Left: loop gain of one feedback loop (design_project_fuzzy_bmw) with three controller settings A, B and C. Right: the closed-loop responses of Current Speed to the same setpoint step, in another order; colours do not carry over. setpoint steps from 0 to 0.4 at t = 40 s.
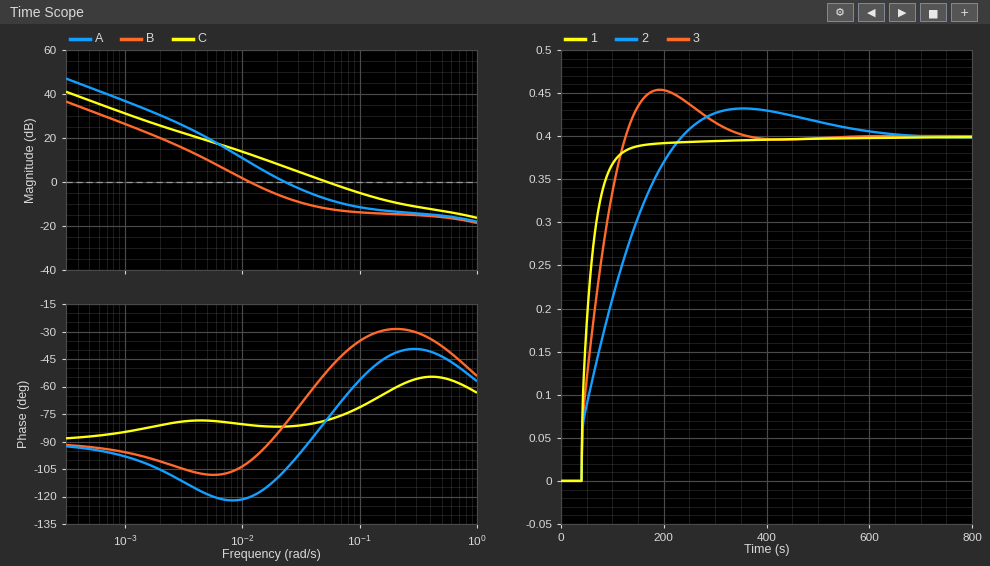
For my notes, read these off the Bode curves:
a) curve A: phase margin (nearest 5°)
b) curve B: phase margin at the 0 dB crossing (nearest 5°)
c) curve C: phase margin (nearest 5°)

75°
80°
100°
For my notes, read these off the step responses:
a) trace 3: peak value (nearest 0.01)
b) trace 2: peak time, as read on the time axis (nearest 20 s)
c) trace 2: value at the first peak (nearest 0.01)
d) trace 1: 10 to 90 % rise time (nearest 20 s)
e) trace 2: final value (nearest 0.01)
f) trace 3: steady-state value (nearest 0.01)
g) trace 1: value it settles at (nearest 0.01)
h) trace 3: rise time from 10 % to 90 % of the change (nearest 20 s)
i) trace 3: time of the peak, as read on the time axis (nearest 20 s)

0.45
360 s
0.43
60 s
0.40
0.40
0.40
60 s
200 s
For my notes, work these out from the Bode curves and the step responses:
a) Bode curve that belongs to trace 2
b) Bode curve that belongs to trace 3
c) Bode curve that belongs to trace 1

B
A
C
